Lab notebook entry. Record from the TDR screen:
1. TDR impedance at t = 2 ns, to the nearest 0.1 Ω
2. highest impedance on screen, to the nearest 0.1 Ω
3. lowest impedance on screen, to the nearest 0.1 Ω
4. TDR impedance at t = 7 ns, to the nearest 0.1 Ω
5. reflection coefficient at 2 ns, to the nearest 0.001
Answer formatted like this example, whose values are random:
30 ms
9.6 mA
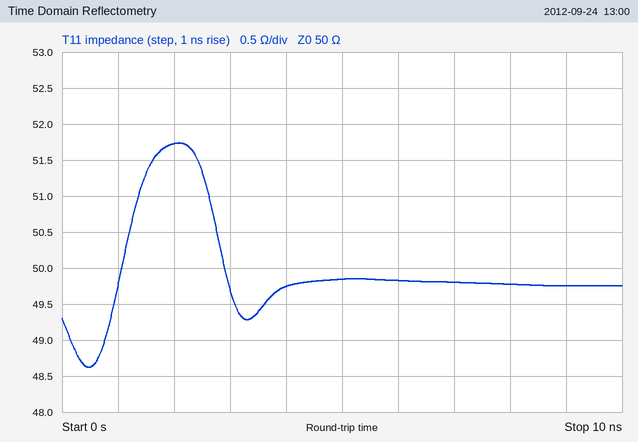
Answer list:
51.7 Ω
51.7 Ω
48.6 Ω
49.8 Ω
+0.017
